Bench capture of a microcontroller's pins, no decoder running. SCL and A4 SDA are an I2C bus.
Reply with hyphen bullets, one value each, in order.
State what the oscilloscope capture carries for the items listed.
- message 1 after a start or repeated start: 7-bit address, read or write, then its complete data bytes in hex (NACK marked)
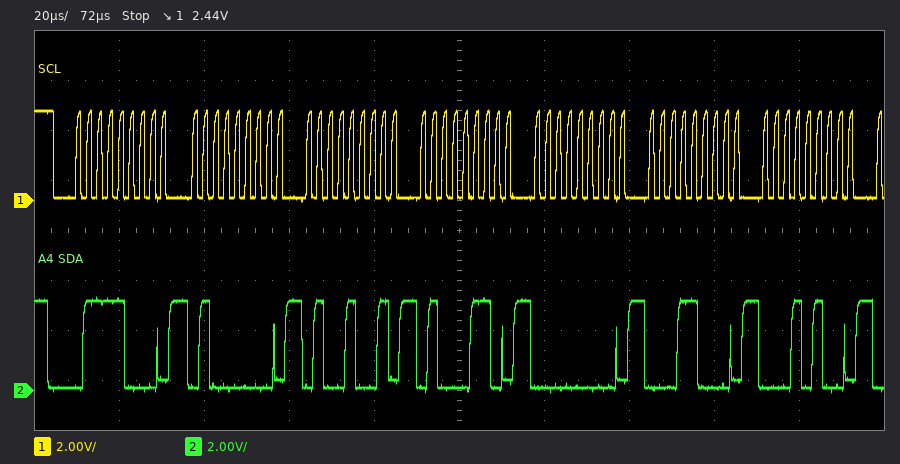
- 0x3C write: 40 49 46 00 18 14
